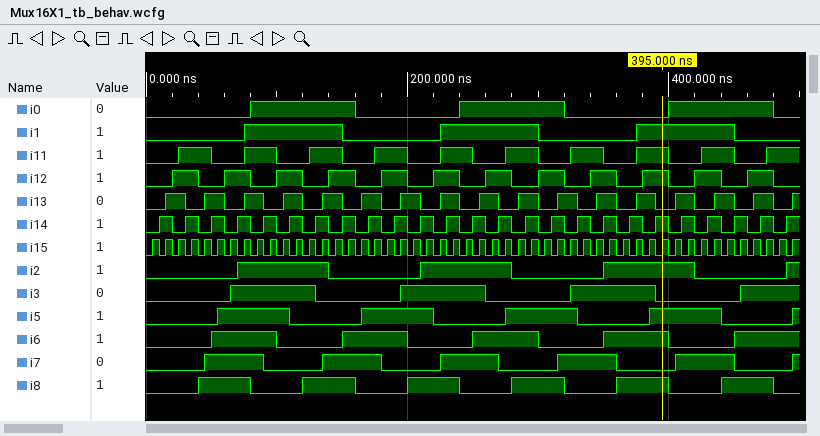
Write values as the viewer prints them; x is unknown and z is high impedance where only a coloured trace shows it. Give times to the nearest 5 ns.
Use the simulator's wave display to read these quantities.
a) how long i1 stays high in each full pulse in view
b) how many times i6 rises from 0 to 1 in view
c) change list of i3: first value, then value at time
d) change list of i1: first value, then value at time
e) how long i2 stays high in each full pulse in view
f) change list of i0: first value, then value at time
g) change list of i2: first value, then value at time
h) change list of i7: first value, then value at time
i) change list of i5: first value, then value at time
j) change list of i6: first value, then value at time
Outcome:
75 ns, 75 ns, 75 ns
5
0, 1 at 65 ns, 0 at 130 ns, 1 at 195 ns, 0 at 260 ns, 1 at 325 ns, 0 at 390 ns, 1 at 455 ns
0, 1 at 75 ns, 0 at 150 ns, 1 at 225 ns, 0 at 300 ns, 1 at 375 ns, 0 at 450 ns
70 ns, 70 ns, 70 ns
0, 1 at 80 ns, 0 at 160 ns, 1 at 240 ns, 0 at 320 ns, 1 at 400 ns, 0 at 480 ns
0, 1 at 70 ns, 0 at 140 ns, 1 at 210 ns, 0 at 280 ns, 1 at 350 ns, 0 at 420 ns, 1 at 490 ns
0, 1 at 45 ns, 0 at 90 ns, 1 at 135 ns, 0 at 180 ns, 1 at 225 ns, 0 at 270 ns, 1 at 315 ns, 0 at 360 ns, 1 at 405 ns, 0 at 450 ns, 1 at 495 ns
0, 1 at 55 ns, 0 at 110 ns, 1 at 165 ns, 0 at 220 ns, 1 at 275 ns, 0 at 330 ns, 1 at 385 ns, 0 at 440 ns, 1 at 495 ns
0, 1 at 50 ns, 0 at 100 ns, 1 at 150 ns, 0 at 200 ns, 1 at 250 ns, 0 at 300 ns, 1 at 350 ns, 0 at 400 ns, 1 at 450 ns
